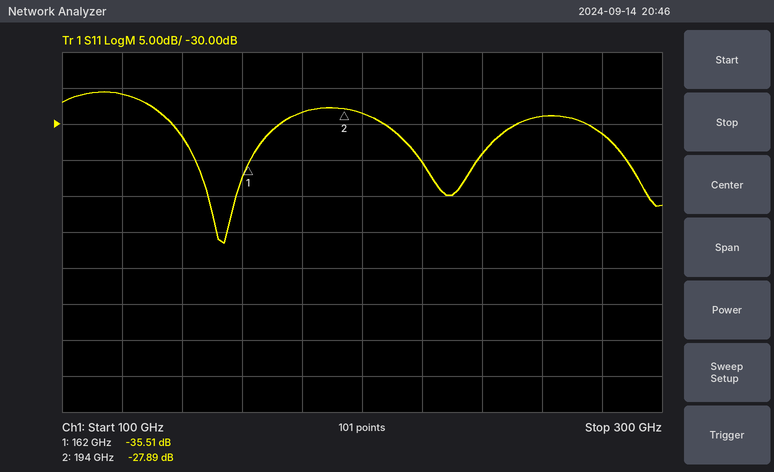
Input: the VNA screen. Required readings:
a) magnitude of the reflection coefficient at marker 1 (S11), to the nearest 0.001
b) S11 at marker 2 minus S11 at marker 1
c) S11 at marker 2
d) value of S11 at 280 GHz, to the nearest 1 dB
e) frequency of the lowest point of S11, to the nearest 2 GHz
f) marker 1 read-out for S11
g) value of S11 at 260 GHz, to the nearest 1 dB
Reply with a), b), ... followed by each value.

a) 0.017
b) 7.62 dB
c) -27.89 dB
d) -31 dB
e) 154 GHz
f) -35.51 dB
g) -29 dB
